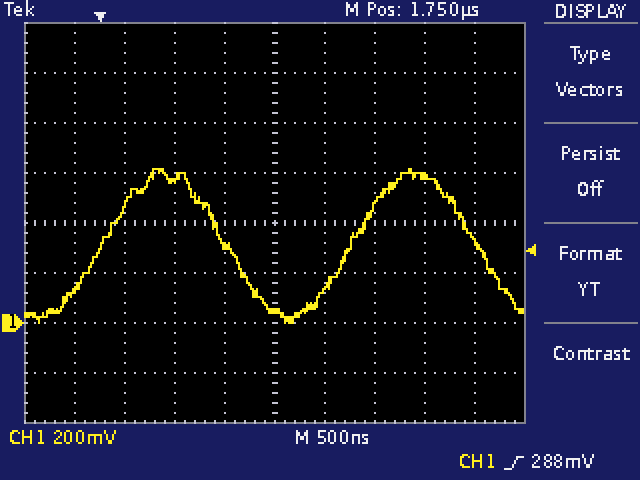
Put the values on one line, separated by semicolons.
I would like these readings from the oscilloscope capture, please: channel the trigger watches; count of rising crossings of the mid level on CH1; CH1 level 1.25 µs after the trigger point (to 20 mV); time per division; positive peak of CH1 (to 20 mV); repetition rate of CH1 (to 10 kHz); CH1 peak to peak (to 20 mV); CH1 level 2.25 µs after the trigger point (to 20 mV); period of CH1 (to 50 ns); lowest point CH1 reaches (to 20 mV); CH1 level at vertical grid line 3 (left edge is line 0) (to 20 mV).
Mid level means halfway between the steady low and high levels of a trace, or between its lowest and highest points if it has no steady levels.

CH1; 2; 320 mV; 500 ns; 620 mV; 400 kHz; 620 mV; 140 mV; 2.50 µs; 0 mV; 580 mV
